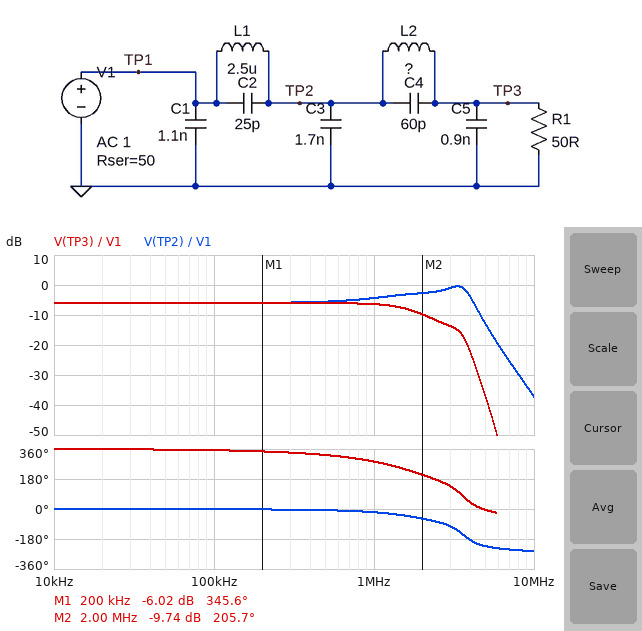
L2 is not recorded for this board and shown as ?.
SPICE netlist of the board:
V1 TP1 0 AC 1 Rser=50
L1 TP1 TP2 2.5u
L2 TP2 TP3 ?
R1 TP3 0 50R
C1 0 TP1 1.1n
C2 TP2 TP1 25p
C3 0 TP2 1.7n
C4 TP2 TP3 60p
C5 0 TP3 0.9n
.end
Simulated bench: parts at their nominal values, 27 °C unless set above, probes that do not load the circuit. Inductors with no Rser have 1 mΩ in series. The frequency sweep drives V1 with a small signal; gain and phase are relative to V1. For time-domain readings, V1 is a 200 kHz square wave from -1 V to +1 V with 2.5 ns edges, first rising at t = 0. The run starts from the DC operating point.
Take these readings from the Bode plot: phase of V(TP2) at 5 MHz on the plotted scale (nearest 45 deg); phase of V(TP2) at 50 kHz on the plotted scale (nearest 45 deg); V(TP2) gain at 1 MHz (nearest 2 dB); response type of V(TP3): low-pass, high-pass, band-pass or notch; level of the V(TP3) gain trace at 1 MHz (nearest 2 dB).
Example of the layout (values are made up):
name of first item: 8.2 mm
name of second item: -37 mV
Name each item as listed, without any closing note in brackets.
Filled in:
phase of V(TP2) at 5 MHz on the plotted scale: -225 deg
phase of V(TP2) at 50 kHz on the plotted scale: 0 deg
V(TP2) gain at 1 MHz: -4 dB
response type of V(TP3): low-pass, high-pass, band-pass or notch: low-pass
level of the V(TP3) gain trace at 1 MHz: -6 dB
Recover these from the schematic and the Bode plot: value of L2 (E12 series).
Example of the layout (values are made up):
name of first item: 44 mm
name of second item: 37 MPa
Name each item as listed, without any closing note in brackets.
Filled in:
value of L2: 8.2 µH
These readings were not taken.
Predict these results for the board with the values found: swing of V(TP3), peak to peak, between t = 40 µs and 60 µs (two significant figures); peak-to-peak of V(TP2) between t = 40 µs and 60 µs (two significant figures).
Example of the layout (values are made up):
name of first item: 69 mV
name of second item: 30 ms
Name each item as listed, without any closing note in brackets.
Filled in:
swing of V(TP3), peak to peak, between t = 40 µs and 60 µs: 1.1 V
peak-to-peak of V(TP2) between t = 40 µs and 60 µs: 2.0 V
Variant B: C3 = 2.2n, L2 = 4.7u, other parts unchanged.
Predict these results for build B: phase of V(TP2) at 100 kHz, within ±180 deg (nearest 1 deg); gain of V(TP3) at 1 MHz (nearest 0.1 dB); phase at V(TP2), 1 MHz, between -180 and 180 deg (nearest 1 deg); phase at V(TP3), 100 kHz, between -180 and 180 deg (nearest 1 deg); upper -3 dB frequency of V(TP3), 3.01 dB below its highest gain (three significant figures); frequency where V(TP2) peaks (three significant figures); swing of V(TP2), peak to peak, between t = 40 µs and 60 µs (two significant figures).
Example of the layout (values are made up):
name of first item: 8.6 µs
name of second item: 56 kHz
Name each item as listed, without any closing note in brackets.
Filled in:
phase of V(TP2) at 100 kHz, within ±180 deg: -3 deg
gain of V(TP3) at 1 MHz: -6.2 dB
phase at V(TP2), 1 MHz, between -180 and 180 deg: -29 deg
phase at V(TP3), 100 kHz, between -180 and 180 deg: -6 deg
upper -3 dB frequency of V(TP3), 3.01 dB below its highest gain: 3.06 MHz
frequency where V(TP2) peaks: 3.22 MHz
swing of V(TP2), peak to peak, between t = 40 µs and 60 µs: 1.5 V
